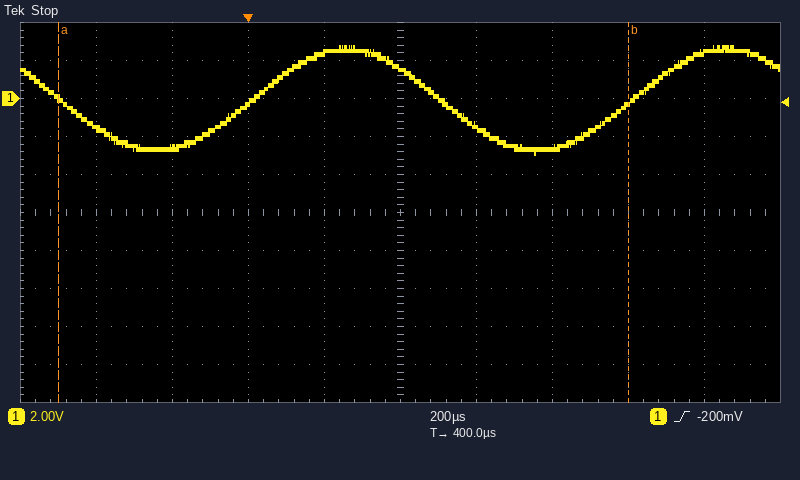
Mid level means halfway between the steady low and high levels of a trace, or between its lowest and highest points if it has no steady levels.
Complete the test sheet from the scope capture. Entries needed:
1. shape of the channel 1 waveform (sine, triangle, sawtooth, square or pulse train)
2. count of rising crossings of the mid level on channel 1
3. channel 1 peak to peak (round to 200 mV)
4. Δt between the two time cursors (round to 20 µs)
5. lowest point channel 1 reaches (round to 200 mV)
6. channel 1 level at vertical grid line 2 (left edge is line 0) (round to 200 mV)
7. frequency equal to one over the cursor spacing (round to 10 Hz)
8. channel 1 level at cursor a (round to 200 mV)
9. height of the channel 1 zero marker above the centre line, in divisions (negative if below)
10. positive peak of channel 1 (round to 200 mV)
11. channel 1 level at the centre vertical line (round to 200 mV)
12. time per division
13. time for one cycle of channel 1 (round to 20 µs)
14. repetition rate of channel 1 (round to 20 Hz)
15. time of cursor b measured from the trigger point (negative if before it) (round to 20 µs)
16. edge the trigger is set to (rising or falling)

sine
2
5.8 V
1.50 ms
-3.0 V
-2.6 V
670 Hz
0.0 V
+3.0 div
2.8 V
1.6 V
200 µs
1.00 ms
1.00 kHz
+1.00 ms
rising
